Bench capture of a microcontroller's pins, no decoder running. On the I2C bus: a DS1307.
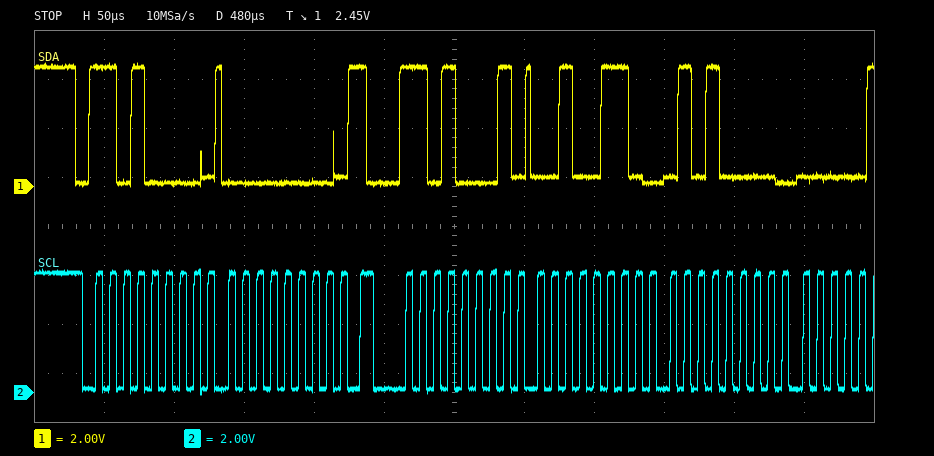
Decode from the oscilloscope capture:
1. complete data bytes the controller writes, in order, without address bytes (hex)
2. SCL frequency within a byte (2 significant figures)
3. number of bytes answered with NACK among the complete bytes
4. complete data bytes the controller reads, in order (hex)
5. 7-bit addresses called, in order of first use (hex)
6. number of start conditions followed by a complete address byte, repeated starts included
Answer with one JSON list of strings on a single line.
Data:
["00", "100 kHz", "0", "26 50", "0x68", "2"]
